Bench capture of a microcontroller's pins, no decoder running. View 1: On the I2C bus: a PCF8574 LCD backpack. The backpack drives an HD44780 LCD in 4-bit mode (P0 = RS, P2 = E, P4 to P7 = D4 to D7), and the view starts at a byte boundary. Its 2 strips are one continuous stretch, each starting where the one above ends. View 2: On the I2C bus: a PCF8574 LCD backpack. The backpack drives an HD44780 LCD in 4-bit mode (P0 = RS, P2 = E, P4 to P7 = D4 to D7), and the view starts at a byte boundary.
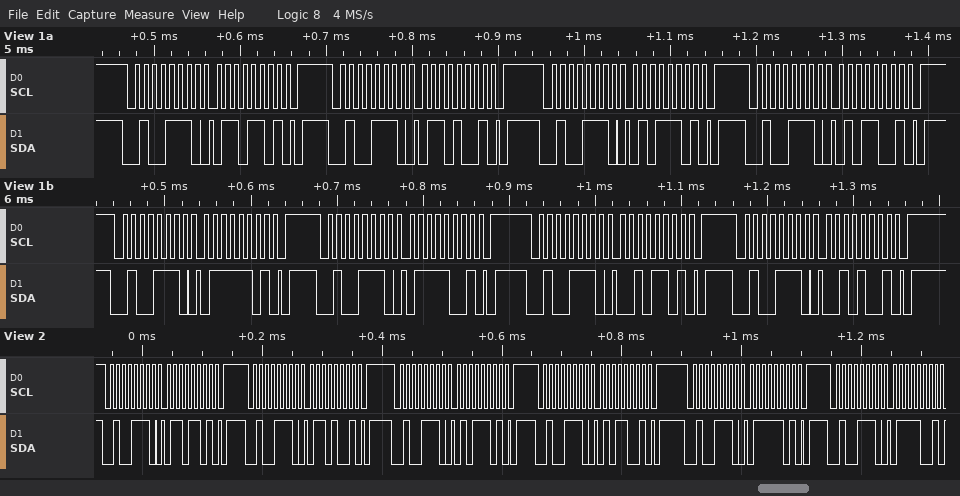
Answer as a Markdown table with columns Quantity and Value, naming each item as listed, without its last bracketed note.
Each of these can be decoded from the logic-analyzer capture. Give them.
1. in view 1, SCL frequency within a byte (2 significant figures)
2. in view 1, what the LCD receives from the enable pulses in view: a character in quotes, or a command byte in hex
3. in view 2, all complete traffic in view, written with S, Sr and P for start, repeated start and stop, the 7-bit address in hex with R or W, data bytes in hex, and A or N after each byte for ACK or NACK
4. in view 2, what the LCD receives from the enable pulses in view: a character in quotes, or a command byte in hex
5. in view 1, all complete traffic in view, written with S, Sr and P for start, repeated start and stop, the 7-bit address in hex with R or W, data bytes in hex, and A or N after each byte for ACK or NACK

| Quantity | Value |
|---|---|
| in view 1, SCL frequency within a byte | 100 kHz |
| in view 1, what the LCD receives from the enable pulses in view: a character in quotes, or a command byte in hex | 'e' 'r' |
| in view 2, all complete traffic in view, written with S, Sr and P for start, repeated start and stop, the 7-bit address in hex with R or W, data bytes in hex, and A or N after each byte for ACK or NACK | S 27W A 6D A P S 27W A 69 A P S 27W A 5D A P S 27W A 59 A P S 27W A 7D A P S 27W A 79 A |
| in view 2, what the LCD receives from the enable pulses in view: a character in quotes, or a command byte in hex | 'e' |
| in view 1, all complete traffic in view, written with S, Sr and P for start, repeated start and stop, the 7-bit address in hex with R or W, data bytes in hex, and A or N after each byte for ACK or NACK | S 27W A 6D A P S 27W A 69 A P S 27W A 5D A P S 27W A 59 A P S 27W A 7D A P S 27W A 79 A P S 27W A 2D A P S 27W A 29 A P |
